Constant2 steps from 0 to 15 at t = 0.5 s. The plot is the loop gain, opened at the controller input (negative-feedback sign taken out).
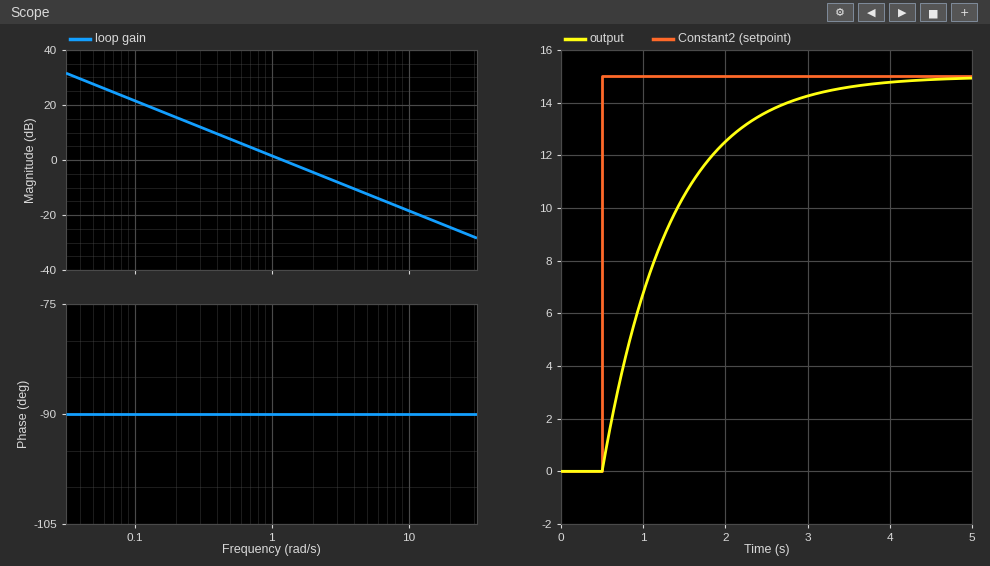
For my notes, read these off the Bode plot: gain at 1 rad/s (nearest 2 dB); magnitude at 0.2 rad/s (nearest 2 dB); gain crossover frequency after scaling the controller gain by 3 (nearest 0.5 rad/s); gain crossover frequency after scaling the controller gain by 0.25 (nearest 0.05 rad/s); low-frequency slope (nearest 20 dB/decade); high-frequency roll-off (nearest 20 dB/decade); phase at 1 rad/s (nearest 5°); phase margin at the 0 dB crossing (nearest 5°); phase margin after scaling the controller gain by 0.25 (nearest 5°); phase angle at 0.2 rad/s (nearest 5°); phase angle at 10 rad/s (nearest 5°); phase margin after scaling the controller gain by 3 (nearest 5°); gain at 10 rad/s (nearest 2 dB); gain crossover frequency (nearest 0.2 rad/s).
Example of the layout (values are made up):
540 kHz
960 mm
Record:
2 dB
16 dB
3.5 rad/s
0.30 rad/s
-20 dB/decade
-20 dB/decade
-90°
90°
90°
-90°
-90°
90°
-18 dB
1.2 rad/s
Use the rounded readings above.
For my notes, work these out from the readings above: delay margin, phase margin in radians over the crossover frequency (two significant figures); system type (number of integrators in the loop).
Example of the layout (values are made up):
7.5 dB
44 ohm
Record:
1.3 s
1
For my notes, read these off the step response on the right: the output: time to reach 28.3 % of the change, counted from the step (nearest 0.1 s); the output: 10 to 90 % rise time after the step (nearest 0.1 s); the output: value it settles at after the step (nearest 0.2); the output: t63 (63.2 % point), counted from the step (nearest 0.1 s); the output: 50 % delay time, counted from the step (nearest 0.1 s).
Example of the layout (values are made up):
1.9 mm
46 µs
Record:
0.3 s
1.8 s
15.0
0.8 s
0.6 s
